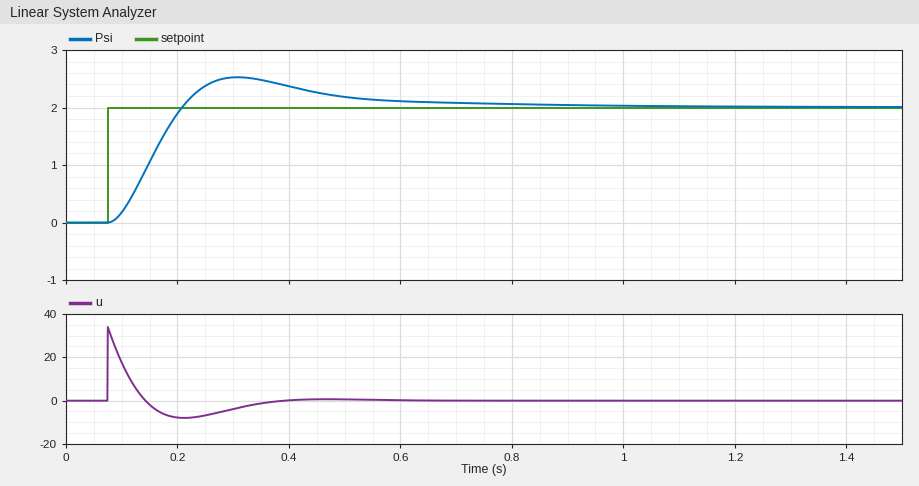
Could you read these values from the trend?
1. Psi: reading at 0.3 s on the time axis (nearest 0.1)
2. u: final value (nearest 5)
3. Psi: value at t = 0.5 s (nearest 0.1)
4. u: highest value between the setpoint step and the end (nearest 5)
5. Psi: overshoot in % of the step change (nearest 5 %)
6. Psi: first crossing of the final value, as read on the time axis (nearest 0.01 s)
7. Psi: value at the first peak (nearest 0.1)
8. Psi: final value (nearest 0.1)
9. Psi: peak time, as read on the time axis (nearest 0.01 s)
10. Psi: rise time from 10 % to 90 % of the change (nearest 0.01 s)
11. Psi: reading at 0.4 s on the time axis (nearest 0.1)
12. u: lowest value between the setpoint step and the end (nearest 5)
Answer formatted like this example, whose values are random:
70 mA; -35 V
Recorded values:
2.5; 0; 2.2; 35; 25 %; 0.21 s; 2.5; 2.0; 0.31 s; 0.09 s; 2.4; -10
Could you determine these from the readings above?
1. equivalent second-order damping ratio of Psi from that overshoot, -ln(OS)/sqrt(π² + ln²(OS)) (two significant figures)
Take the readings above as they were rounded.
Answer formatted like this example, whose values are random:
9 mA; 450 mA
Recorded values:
0.40
